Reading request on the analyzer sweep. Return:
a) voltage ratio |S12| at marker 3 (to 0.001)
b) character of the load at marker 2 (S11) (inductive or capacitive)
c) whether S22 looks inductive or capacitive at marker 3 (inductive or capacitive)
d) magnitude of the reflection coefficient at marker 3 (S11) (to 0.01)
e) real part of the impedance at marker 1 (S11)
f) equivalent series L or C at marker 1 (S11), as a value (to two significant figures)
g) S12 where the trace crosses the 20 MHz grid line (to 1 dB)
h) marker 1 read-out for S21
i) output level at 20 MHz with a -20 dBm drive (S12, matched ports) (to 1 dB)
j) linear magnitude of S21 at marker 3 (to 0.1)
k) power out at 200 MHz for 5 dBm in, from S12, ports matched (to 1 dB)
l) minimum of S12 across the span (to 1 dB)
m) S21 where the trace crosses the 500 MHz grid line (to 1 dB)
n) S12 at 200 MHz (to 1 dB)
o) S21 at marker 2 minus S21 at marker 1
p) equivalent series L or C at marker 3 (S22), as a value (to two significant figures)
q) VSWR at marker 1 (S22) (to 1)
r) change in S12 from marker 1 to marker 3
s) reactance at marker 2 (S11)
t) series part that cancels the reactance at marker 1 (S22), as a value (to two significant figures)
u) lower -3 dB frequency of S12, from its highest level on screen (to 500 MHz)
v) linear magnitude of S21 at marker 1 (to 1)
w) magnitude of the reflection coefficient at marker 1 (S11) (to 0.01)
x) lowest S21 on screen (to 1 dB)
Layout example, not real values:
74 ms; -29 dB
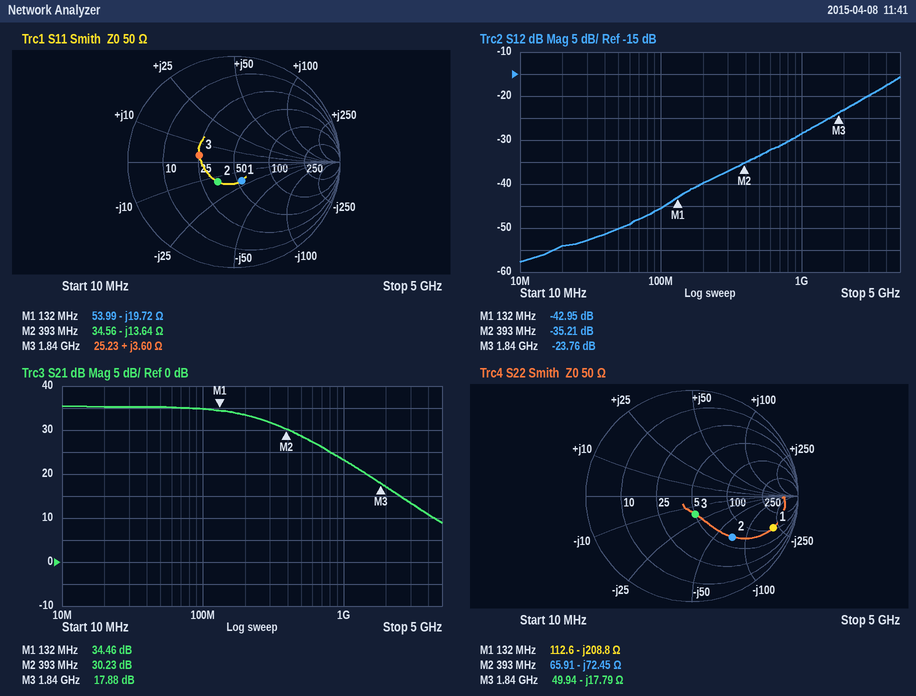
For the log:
0.065; capacitive; capacitive; 0.33; 53.99 Ω; 61 pF; -54 dB; 34.46 dB; -74 dBm; 7.8; -35 dBm; -58 dB; 29 dB; -40 dB; -4.23 dB; 4.9 pF; 10; 19.19 dB; -13.64 Ω; 250 nH; 3.5 GHz; 53; 0.19; 9 dB
